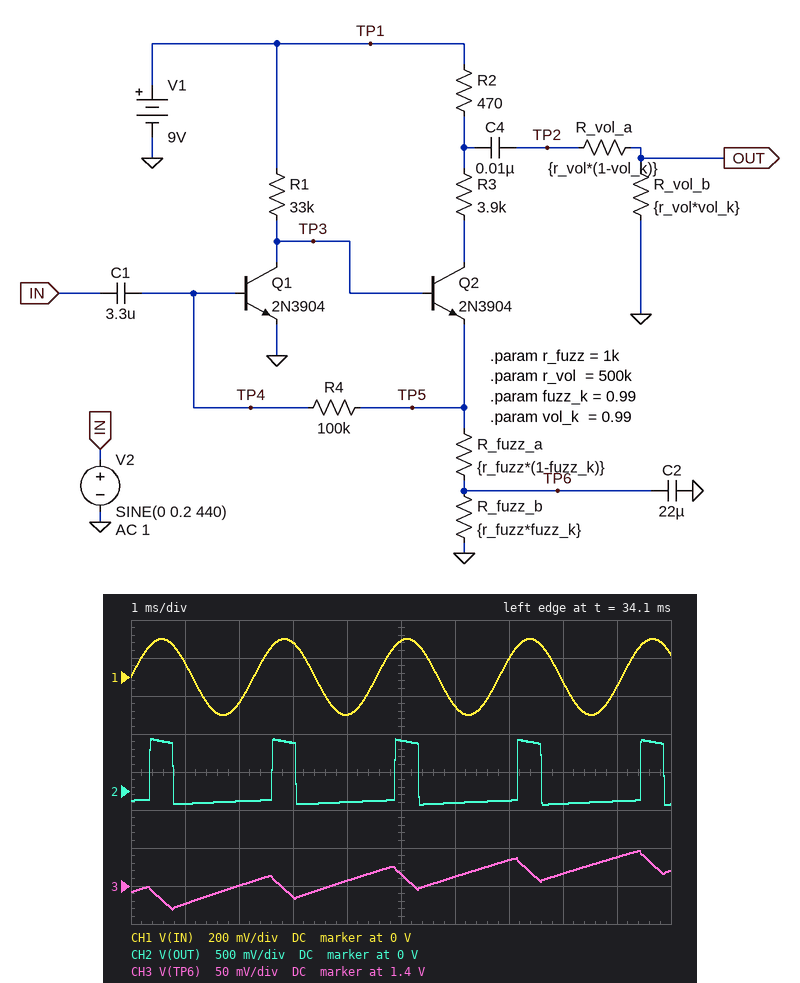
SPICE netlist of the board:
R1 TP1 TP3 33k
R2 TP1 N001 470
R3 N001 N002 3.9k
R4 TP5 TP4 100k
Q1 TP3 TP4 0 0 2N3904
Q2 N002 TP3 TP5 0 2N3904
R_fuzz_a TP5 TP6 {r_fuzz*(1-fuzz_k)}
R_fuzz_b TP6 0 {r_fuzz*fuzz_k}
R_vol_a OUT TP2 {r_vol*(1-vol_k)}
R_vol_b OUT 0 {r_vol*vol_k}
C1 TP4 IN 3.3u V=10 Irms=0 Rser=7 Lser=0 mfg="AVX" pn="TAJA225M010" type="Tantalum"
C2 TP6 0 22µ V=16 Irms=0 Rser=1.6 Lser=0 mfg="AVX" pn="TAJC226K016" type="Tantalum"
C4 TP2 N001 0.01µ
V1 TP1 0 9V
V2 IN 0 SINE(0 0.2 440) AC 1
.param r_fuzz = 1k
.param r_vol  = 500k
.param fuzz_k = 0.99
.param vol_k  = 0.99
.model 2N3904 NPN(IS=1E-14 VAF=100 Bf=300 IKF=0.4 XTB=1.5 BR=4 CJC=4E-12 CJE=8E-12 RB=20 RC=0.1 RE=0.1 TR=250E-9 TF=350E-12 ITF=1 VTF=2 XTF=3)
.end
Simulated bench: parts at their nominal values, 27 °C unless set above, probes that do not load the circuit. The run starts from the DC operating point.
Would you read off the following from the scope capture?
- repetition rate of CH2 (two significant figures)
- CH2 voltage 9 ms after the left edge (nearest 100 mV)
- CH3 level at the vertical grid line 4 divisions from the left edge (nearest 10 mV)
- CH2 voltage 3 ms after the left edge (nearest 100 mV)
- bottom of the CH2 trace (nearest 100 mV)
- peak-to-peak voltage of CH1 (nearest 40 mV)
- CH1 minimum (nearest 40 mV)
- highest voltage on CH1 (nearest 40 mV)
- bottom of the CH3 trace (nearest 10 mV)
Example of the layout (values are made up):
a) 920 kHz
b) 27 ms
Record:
a) 440 Hz
b) -100 mV
c) 1.41 V
d) 600 mV
e) -200 mV
f) 400 mV
g) -200 mV
h) 200 mV
i) 1.37 V
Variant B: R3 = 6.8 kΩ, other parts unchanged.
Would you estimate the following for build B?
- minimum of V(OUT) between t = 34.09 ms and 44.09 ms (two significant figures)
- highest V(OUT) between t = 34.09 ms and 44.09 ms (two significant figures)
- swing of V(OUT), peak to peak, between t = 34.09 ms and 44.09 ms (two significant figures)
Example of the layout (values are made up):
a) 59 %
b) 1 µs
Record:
a) -98 mV
b) 440 mV
c) 540 mV
